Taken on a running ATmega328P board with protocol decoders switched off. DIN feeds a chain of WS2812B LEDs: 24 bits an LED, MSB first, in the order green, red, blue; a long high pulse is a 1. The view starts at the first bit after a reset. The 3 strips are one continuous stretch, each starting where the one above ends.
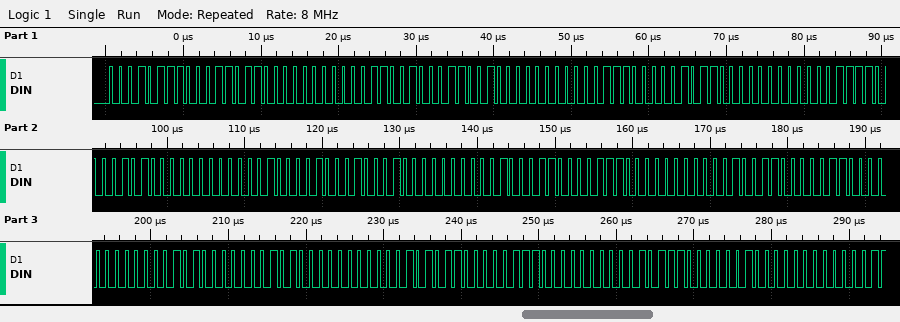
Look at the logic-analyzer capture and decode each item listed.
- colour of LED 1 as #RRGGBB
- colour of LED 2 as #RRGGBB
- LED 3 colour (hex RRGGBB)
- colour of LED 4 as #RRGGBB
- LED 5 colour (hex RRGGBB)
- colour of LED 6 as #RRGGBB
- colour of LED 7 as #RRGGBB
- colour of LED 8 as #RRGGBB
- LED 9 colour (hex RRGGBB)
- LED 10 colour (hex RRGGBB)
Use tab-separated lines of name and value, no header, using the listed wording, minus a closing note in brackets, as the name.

colour of LED 1 as #RRGGBB	#1B1700
colour of LED 2 as #RRGGBB	#191900
LED 3 colour	#161C00
colour of LED 4 as #RRGGBB	#141E00
LED 5 colour	#112100
colour of LED 6 as #RRGGBB	#0E2300
colour of LED 7 as #RRGGBB	#0C2600
colour of LED 8 as #RRGGBB	#0A2800
LED 9 colour	#072B00
LED 10 colour	#042E00
